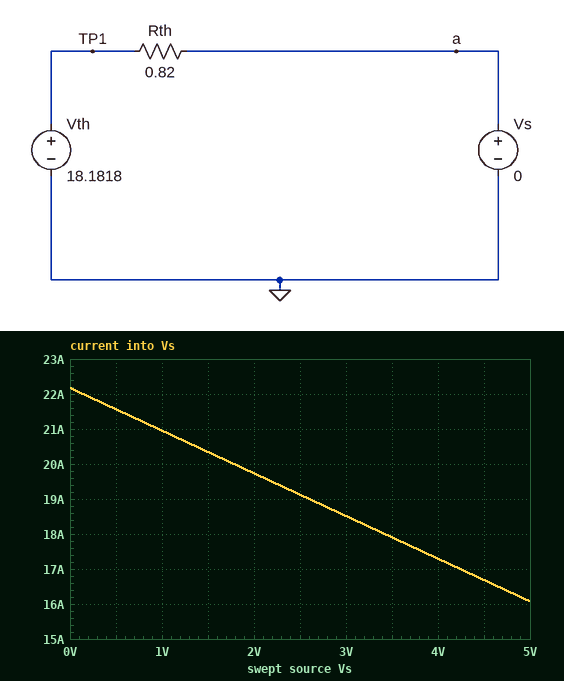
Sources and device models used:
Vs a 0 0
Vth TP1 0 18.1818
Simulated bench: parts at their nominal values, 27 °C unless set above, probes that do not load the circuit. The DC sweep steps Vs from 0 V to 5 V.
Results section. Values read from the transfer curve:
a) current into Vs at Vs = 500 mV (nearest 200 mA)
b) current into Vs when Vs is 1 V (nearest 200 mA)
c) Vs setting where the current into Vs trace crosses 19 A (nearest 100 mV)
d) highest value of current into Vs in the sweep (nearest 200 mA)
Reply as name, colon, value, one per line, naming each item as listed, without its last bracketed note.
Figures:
current into Vs at Vs = 500 mV: 21.6 A
current into Vs when Vs is 1 V: 21.0 A
Vs setting where the current into Vs trace crosses 19 A: 2.6 V
highest value of current into Vs in the sweep: 22.2 A
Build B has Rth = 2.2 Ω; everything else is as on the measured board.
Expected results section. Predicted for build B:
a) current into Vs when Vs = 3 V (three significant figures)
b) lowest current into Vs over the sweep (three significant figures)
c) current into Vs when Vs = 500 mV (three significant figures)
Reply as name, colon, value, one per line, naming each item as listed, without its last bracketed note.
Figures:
current into Vs when Vs = 3 V: 6.90 A
lowest current into Vs over the sweep: 5.99 A
current into Vs when Vs = 500 mV: 8.04 A
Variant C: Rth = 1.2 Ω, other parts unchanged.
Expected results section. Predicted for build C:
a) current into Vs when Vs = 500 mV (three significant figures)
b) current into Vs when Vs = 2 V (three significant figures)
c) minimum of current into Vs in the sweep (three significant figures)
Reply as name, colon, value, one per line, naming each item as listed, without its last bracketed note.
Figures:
current into Vs when Vs = 500 mV: 14.7 A
current into Vs when Vs = 2 V: 13.5 A
minimum of current into Vs in the sweep: 11.0 A
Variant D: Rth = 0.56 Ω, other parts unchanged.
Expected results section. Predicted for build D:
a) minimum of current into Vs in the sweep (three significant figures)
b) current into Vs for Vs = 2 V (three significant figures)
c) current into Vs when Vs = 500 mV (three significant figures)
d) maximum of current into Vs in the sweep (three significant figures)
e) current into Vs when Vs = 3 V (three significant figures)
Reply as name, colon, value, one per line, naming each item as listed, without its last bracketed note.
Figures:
minimum of current into Vs in the sweep: 23.5 A
current into Vs for Vs = 2 V: 28.9 A
current into Vs when Vs = 500 mV: 31.6 A
maximum of current into Vs in the sweep: 32.5 A
current into Vs when Vs = 3 V: 27.1 A
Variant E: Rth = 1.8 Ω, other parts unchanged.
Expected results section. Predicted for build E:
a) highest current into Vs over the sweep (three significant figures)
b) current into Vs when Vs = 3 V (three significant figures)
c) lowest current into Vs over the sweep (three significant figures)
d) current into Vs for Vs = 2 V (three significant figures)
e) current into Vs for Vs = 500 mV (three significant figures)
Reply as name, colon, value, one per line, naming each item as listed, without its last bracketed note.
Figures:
highest current into Vs over the sweep: 10.1 A
current into Vs when Vs = 3 V: 8.43 A
lowest current into Vs over the sweep: 7.32 A
current into Vs for Vs = 2 V: 8.99 A
current into Vs for Vs = 500 mV: 9.82 A
